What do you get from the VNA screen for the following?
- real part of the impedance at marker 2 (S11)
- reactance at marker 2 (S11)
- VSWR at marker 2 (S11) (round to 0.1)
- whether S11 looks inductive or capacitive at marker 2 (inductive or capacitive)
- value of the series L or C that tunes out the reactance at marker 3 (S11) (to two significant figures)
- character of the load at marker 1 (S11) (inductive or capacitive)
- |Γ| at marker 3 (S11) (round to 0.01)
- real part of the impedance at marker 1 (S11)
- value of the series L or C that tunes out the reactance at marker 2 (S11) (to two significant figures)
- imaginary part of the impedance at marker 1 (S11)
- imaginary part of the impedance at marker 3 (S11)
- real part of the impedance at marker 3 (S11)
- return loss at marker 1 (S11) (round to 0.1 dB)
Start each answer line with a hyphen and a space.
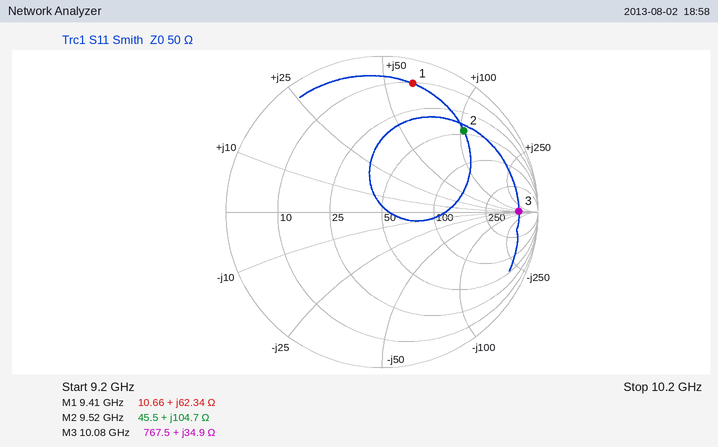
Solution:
- 45.5 Ω
- +104.7 Ω
- 6.7
- inductive
- 450 fF
- inductive
- 0.88
- 10.66 Ω
- 160 fF
- +62.34 Ω
- +34.9 Ω
- 767.5 Ω
- 1.4 dB
